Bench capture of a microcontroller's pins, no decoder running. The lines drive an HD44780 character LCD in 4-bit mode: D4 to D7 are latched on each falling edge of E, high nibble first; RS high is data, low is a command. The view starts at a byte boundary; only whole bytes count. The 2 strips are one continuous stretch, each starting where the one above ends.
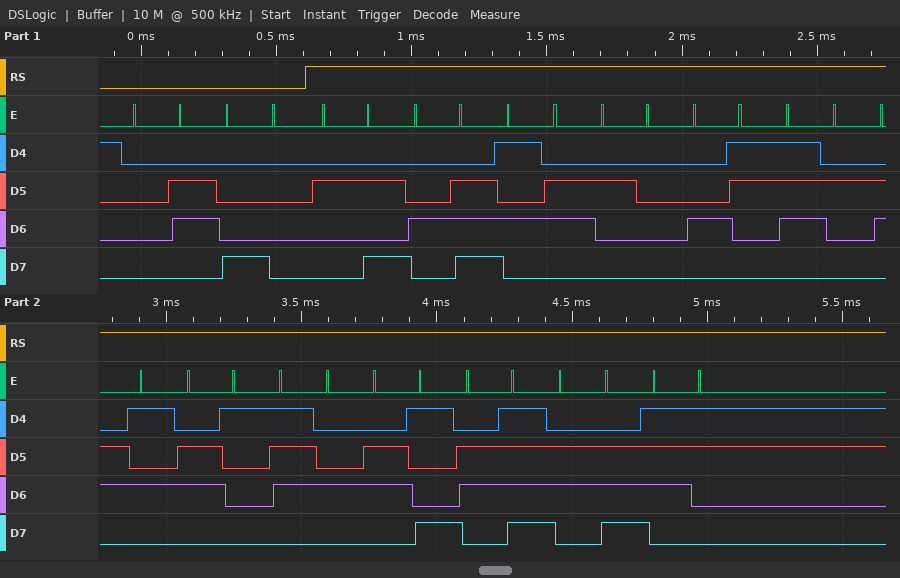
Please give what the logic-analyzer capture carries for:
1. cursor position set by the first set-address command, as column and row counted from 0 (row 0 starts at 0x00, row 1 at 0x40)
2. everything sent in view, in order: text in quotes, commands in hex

column 0, row 0
0x06 0x80 "*NV Creations"
